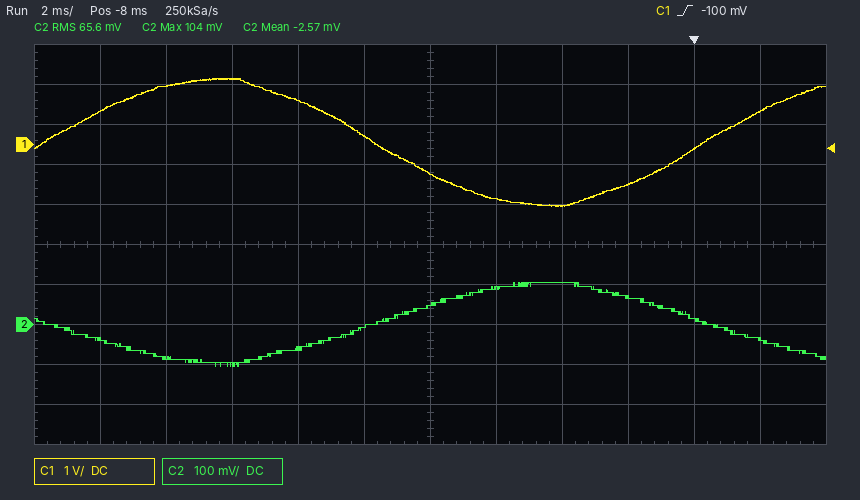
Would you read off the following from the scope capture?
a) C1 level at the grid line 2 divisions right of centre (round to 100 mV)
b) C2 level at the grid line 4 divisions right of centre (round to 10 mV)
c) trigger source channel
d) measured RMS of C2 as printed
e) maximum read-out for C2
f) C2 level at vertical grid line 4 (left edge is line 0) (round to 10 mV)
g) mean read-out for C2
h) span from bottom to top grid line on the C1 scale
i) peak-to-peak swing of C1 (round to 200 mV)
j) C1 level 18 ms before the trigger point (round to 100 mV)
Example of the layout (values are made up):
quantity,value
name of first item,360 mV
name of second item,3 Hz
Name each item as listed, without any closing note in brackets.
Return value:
quantity,value
C1 level at the grid line 2 divisions right of centre,-1.5 V
C2 level at the grid line 4 divisions right of centre,10 mV
trigger source channel,C1
measured RMS of C2 as printed,65.6 mV
maximum read-out for C2,104 mV
C2 level at vertical grid line 4 (left edge is line 0),-60 mV
mean read-out for C2,-2.57 mV
span from bottom to top grid line on the C1 scale,10 V
peak-to-peak swing of C1,3.2 V
C1 level 18 ms before the trigger point,800 mV
